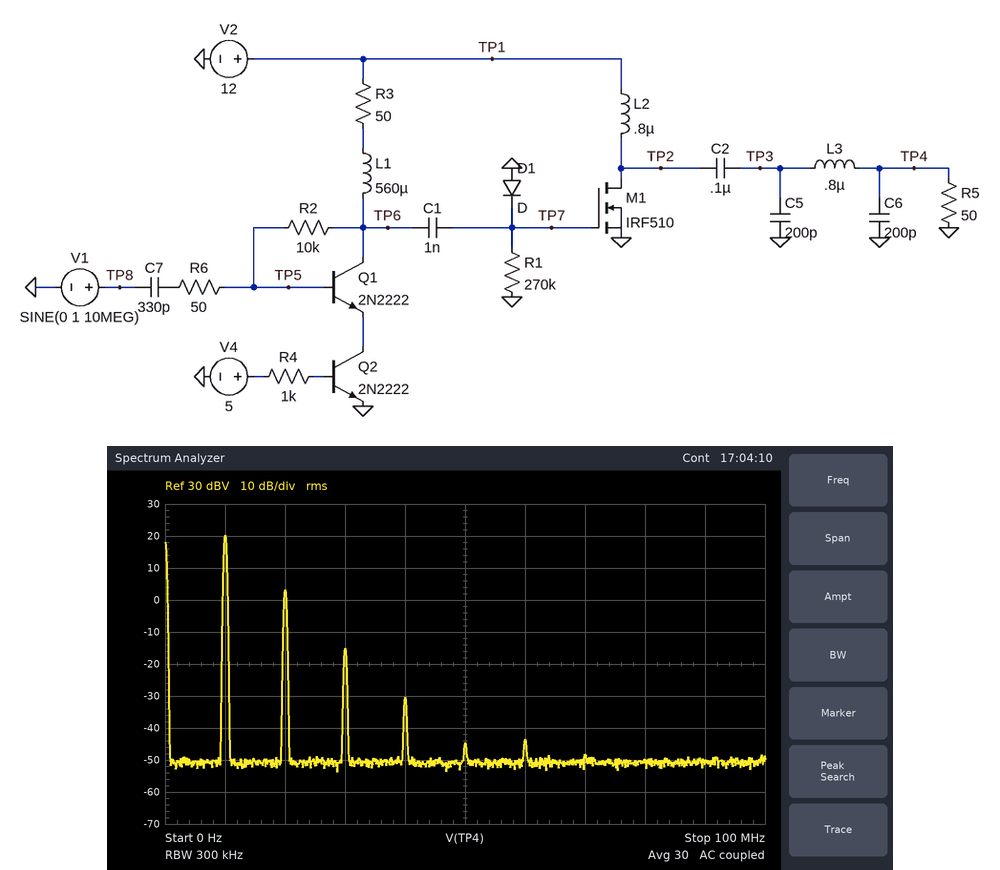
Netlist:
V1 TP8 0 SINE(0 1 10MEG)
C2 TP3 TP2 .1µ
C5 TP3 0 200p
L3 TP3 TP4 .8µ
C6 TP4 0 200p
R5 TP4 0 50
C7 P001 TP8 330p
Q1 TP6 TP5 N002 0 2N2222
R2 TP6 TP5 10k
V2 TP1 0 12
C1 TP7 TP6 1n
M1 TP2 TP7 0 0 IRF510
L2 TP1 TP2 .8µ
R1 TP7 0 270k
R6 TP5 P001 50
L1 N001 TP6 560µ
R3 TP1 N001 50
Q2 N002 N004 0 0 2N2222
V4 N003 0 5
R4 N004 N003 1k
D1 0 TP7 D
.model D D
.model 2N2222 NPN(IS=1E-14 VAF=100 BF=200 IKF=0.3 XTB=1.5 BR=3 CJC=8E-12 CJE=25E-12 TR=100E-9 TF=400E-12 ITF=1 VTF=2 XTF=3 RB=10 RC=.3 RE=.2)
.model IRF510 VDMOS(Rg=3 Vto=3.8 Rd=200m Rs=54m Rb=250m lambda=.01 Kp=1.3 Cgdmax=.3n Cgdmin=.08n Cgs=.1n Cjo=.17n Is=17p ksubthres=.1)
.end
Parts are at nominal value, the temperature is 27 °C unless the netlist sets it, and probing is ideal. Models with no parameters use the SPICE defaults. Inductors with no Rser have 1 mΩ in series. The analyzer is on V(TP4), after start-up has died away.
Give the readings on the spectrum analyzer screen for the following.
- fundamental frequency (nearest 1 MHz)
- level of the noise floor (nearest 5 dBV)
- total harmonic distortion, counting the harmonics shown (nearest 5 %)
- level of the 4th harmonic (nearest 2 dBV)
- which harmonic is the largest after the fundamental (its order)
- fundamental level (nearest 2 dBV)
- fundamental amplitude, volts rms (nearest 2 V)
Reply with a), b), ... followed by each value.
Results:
a) 10 MHz
b) -50 dBV
c) 15 %
d) -30 dBV
e) 2
f) 20 dBV
g) 10 V
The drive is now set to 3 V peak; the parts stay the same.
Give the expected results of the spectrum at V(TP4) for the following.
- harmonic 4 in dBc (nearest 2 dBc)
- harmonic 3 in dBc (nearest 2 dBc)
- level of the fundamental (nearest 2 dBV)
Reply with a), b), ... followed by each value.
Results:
a) -40 dBc
b) -30 dBc
c) 20 dBV
